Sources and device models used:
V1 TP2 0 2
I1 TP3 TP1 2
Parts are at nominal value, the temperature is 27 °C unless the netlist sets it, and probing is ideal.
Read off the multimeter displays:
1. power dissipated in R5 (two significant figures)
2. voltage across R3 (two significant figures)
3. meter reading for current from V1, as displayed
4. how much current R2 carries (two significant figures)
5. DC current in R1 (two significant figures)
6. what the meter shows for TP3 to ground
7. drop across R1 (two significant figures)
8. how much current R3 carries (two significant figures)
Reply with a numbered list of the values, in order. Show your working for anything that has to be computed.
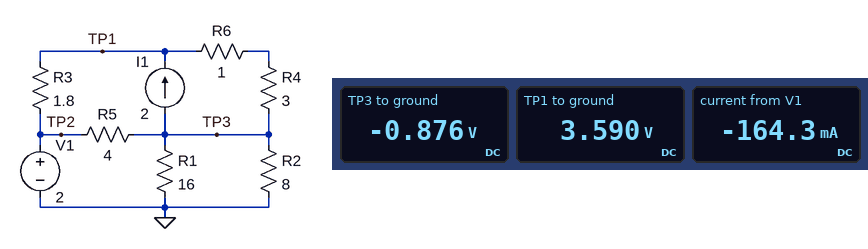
1. (2 V - (-876 mV))^2 / 4 Ω = 2.1 W
2. 3.59 V - 2 V = 1.6 V
3. -164.3 mA
4. (0 V - (-876 mV)) / 8 Ω = 110 mA
5. (0 V - (-876 mV)) / 16 Ω = 55 mA
6. -0.876 V
7. 0 V - (-876 mV) = 880 mV
8. (3.59 V - 2 V) / 1.8 Ω = 880 mA
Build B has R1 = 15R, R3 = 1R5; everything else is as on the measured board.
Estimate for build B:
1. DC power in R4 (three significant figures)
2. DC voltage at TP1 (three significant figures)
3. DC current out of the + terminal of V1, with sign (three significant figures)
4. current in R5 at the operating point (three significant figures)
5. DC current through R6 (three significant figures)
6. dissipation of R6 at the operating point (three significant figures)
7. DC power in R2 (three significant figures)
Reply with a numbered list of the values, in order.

1. 3.51 W
2. 3.38 V
3. -182 mA
4. 737 mA
5. 1.08 A
6. 1.17 W
7. 112 mW
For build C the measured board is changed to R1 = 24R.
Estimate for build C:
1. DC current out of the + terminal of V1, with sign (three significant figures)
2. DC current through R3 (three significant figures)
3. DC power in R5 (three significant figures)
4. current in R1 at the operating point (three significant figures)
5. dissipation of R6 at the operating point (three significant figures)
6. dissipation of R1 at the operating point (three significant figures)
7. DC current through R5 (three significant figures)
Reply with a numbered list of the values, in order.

1. -151 mA
2. 878 mA
3. 2.11 W
4. 37.8 mA
5. 1.26 W
6. 34.3 mW
7. 727 mA
